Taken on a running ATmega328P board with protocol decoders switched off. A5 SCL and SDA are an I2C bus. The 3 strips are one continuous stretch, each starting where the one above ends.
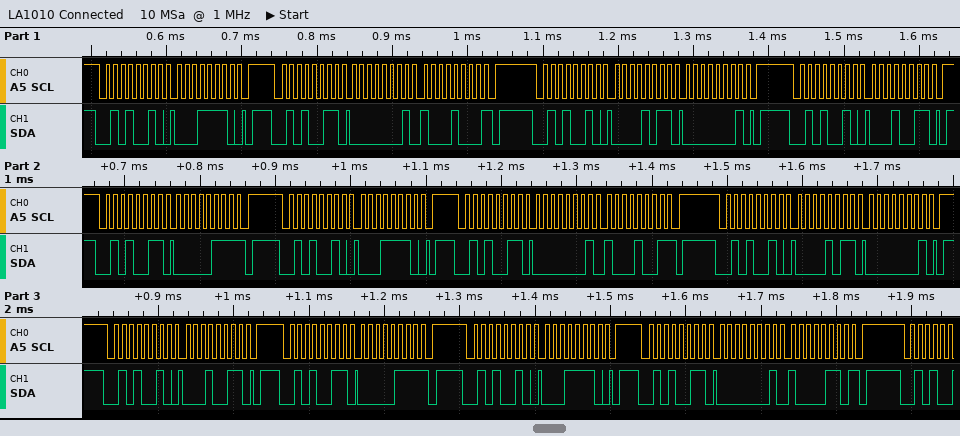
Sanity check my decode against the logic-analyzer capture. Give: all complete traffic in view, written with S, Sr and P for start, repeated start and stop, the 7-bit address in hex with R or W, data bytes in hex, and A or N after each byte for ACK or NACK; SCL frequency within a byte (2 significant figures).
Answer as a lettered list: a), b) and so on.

a) S 29W A 1E A P S 29R A 01 A 88 N P S 29W A 0B A 01 A P S 29W A 13 A P S 29R A 07 N P S 29W A 1E A P S 29R A 01 A 89 N P S 29W A 0B A 01 A P S 29W A 13 A P S 29R A 07 N P S 29W A 1E A P S 29R A 01 A 86 N P
b) 100 kHz
